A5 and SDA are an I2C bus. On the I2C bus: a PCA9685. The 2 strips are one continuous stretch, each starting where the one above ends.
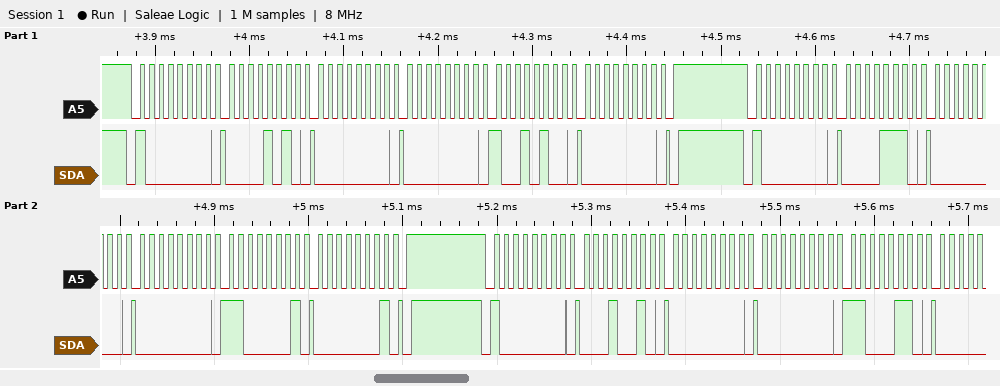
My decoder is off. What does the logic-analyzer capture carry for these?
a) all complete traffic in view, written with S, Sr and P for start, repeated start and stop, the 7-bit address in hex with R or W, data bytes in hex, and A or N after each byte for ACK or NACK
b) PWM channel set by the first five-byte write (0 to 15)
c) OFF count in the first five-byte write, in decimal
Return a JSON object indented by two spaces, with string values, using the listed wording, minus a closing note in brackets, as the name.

{
  "all complete traffic in view, written with S, Sr and P for start, repeated start and stop, the 7-bit address in hex with R or W, data bytes in hex, and A or N after each byte for ACK or NACK": "S 40W A 0A A 00 A 00 A 94 A 00 A P S 40W A 0E A 00 A 00 A C1 A 01 A P S 40W A 12 A 00 A 00 A C6 A",
  "PWM channel set by the first five-byte write": "1",
  "OFF count in the first five-byte write, in decimal": "148"
}
